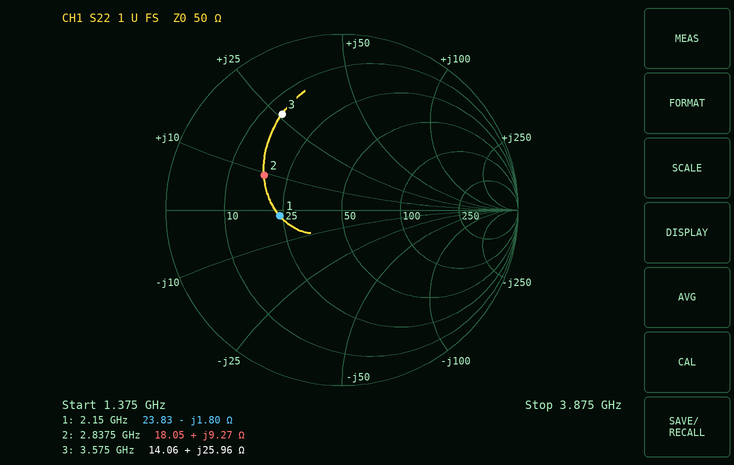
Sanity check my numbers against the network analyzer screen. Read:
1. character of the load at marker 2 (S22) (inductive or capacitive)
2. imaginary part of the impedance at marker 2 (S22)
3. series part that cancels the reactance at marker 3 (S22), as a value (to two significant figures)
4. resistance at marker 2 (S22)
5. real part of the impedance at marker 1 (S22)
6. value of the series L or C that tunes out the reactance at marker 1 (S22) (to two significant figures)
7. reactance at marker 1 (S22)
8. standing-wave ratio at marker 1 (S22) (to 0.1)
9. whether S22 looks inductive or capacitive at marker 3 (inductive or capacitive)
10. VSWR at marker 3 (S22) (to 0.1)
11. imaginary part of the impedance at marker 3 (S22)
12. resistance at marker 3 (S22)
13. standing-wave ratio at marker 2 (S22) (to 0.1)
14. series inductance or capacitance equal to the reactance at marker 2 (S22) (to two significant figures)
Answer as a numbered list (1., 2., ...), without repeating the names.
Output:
1. inductive
2. +9.27 Ω
3. 1.7 pF
4. 18.05 Ω
5. 23.83 Ω
6. 130 pH
7. -1.80 Ω
8. 2.1
9. inductive
10. 4.6
11. +25.96 Ω
12. 14.06 Ω
13. 2.9
14. 520 pH
